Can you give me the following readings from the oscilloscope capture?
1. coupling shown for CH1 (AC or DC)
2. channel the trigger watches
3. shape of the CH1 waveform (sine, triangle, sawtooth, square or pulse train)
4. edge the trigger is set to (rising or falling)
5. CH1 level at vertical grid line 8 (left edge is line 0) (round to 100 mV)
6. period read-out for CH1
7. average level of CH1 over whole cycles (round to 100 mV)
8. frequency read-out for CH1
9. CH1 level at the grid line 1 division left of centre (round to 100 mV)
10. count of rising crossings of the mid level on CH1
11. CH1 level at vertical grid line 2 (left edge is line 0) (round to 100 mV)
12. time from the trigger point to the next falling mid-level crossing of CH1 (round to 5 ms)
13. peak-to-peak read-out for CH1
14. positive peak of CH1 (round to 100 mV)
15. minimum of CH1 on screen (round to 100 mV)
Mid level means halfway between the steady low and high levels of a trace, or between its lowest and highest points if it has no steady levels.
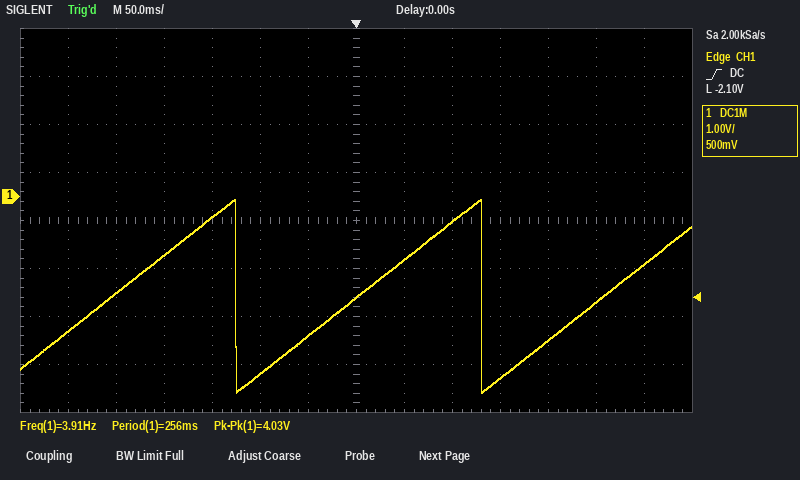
DC
CH1
sawtooth
rising
-1.3 V
256 ms
-2.1 V
3.91 Hz
-2.9 V
3
-2.0 V
130 ms
4.03 V
-100 mV
-4.1 V
